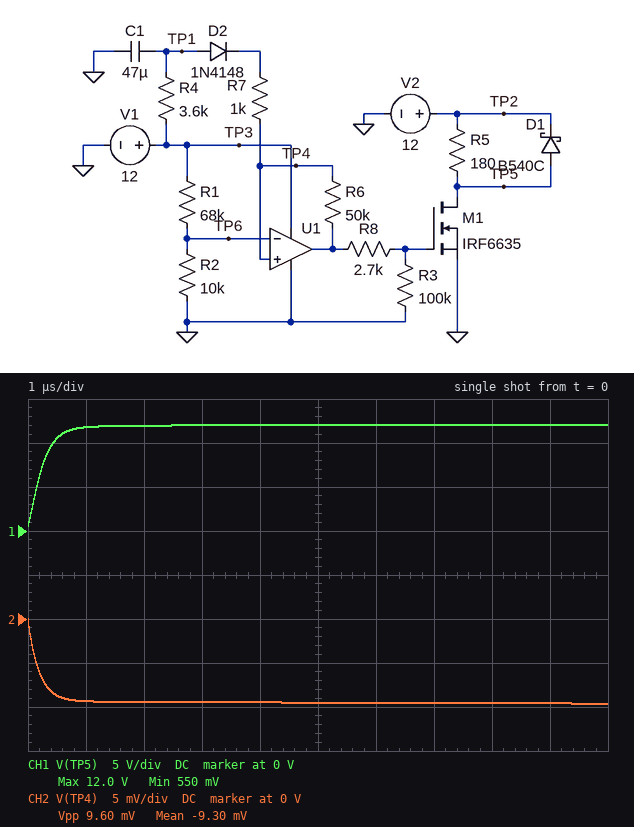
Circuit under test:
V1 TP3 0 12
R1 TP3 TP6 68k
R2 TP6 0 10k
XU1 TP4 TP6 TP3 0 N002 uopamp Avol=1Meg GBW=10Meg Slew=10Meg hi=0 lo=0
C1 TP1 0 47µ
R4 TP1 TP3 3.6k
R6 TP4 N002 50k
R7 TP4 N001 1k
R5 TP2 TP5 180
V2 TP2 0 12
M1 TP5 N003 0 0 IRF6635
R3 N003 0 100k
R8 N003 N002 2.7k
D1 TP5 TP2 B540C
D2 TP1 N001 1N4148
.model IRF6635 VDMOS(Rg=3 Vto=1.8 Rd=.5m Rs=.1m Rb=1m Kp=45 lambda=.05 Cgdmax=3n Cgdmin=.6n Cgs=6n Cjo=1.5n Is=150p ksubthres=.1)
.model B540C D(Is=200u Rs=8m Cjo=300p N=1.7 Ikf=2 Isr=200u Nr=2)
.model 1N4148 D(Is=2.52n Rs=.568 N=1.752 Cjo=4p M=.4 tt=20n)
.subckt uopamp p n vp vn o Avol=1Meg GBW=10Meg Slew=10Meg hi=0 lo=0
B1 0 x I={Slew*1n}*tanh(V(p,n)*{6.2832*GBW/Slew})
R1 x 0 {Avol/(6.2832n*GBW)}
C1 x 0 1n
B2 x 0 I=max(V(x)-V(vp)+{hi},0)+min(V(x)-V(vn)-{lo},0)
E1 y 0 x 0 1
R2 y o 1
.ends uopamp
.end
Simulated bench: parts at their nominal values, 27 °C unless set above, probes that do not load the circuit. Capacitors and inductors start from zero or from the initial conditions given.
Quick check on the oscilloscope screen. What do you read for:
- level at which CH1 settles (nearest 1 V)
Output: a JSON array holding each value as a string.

["12 V"]
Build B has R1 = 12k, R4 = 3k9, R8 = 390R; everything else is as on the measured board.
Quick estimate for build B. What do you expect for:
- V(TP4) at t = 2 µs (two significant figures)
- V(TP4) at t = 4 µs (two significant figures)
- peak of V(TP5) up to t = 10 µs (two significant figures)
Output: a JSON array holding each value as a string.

["-7.8 mV", "-8.9 mV", "12 V"]
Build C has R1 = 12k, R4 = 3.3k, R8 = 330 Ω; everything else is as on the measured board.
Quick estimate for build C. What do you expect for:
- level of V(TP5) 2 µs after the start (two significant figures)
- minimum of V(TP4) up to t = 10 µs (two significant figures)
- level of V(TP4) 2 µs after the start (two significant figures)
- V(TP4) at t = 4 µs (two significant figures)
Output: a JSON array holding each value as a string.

["12 V", "-9.9 mV", "-7.6 mV", "-9.0 mV"]
